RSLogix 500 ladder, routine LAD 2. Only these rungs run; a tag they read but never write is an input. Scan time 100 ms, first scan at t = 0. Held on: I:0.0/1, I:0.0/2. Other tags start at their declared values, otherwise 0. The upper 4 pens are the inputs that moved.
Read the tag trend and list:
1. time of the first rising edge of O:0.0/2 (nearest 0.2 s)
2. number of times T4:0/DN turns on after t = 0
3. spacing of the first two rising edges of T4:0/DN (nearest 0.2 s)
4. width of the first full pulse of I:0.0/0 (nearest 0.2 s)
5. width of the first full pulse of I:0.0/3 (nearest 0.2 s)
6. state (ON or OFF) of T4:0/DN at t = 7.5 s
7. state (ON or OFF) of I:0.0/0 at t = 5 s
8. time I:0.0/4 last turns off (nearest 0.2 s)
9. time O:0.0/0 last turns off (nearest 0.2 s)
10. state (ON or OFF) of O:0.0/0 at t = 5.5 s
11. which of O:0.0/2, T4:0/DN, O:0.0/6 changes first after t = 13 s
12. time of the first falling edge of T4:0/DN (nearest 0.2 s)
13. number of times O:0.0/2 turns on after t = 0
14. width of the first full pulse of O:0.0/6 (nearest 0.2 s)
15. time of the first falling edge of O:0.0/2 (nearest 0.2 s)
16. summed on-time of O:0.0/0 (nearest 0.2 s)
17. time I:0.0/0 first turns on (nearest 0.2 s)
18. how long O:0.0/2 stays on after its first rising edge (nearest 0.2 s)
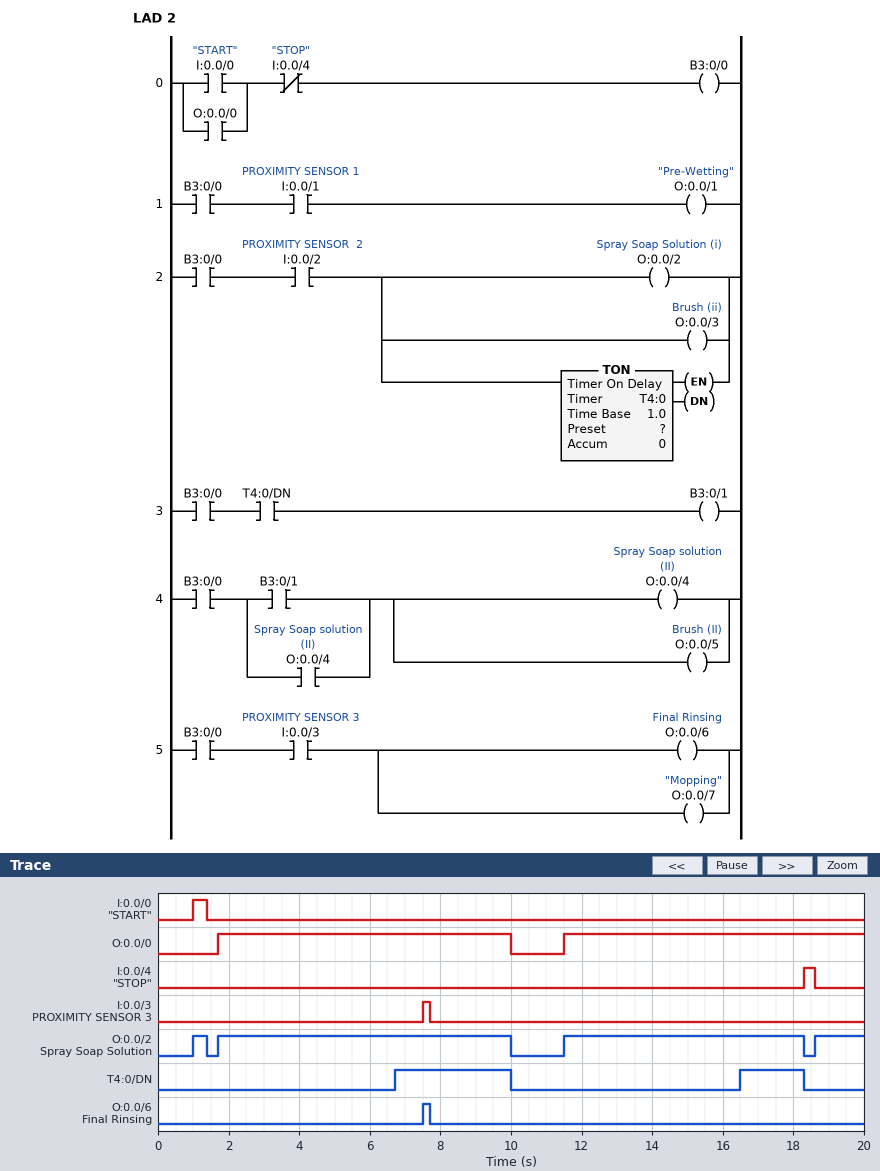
1.0 s
2
9.8 s
0.4 s
0.2 s
ON
OFF
18.6 s
10.0 s
ON
T4:0/DN
10.0 s
4
0.2 s
1.4 s
16.8 s
1.0 s
0.4 s
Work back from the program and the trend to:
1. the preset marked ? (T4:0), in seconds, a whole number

5 s
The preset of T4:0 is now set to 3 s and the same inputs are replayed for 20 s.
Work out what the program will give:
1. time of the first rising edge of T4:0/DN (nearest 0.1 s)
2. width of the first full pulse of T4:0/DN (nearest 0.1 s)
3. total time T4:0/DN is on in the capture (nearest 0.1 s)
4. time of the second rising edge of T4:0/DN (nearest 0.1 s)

4.7 s
5.3 s
9.1 s
14.5 s
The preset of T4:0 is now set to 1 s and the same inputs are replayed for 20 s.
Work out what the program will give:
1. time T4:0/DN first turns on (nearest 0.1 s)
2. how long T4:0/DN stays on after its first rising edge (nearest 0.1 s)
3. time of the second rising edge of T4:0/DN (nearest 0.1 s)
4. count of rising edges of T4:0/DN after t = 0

2.7 s
7.3 s
12.5 s
3
